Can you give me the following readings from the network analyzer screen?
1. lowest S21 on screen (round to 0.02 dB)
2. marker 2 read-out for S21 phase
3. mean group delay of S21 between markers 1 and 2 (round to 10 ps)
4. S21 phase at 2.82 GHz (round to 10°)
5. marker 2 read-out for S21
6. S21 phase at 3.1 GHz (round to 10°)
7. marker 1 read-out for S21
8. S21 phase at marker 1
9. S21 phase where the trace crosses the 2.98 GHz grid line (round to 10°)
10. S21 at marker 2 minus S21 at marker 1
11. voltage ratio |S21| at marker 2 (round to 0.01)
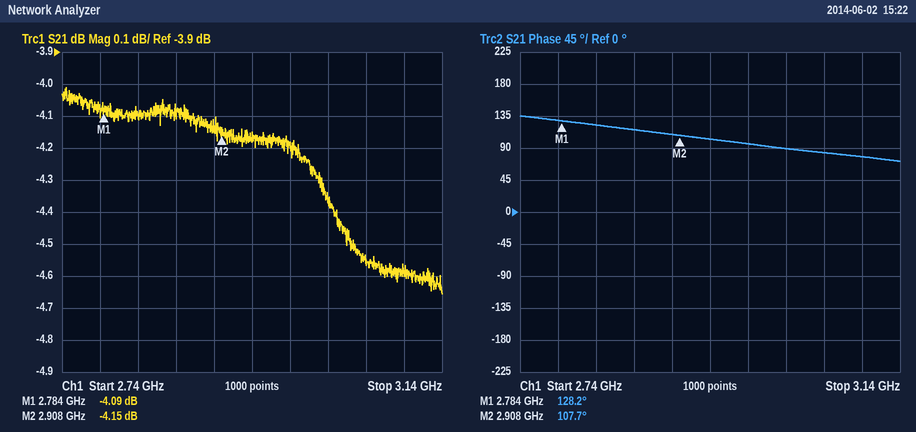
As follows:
-4.66 dB
107.7°
460 ps
120°
-4.15 dB
80°
-4.09 dB
128.2°
100°
-0.06 dB
0.62
